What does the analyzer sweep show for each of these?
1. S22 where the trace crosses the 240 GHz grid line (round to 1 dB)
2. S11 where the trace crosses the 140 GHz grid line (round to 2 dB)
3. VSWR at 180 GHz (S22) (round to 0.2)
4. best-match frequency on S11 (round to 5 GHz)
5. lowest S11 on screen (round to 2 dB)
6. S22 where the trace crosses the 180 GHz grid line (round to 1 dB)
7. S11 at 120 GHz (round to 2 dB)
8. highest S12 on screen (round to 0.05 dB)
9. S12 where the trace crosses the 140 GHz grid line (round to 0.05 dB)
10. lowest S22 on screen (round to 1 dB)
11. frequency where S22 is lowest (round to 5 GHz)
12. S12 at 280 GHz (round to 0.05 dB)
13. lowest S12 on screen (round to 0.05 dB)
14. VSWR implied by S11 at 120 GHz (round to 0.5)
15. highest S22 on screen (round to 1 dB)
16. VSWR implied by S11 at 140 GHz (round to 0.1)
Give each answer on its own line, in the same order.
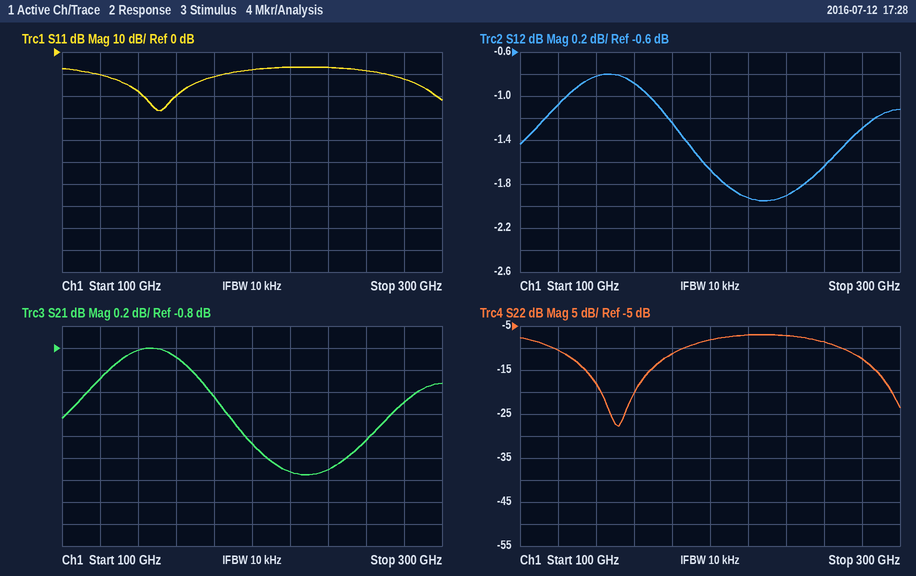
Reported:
-7 dB
-18 dB
1.8
150 GHz
-26 dB
-11 dB
-10 dB
-0.80 dB
-0.80 dB
-28 dB
150 GHz
-1.30 dB
-1.95 dB
2.0
-7 dB
1.3
